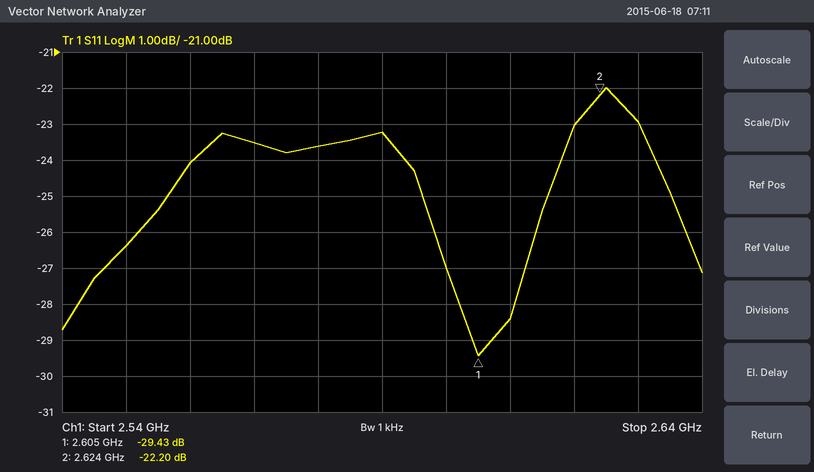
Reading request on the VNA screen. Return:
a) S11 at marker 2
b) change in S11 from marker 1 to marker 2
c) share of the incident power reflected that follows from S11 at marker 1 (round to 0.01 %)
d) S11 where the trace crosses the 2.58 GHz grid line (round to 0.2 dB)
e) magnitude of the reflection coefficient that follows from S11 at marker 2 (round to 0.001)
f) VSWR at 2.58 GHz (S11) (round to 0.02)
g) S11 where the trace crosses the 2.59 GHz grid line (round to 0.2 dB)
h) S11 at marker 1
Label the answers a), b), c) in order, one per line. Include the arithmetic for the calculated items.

a) -22.20 dB
b) -22.2 − (-29.43) = 7.23 dB
c) 10^(-29.43/10) ≈ 0.11 %
d) -23.6 dB
e) 10^(-22.2/20) ≈ 0.078
f) |Γ| = 10^(-23.6/20) = 0.0661; VSWR = (1 + 0.0661)/(1 − 0.0661) ≈ 1.14
g) -23.2 dB
h) -29.43 dB
